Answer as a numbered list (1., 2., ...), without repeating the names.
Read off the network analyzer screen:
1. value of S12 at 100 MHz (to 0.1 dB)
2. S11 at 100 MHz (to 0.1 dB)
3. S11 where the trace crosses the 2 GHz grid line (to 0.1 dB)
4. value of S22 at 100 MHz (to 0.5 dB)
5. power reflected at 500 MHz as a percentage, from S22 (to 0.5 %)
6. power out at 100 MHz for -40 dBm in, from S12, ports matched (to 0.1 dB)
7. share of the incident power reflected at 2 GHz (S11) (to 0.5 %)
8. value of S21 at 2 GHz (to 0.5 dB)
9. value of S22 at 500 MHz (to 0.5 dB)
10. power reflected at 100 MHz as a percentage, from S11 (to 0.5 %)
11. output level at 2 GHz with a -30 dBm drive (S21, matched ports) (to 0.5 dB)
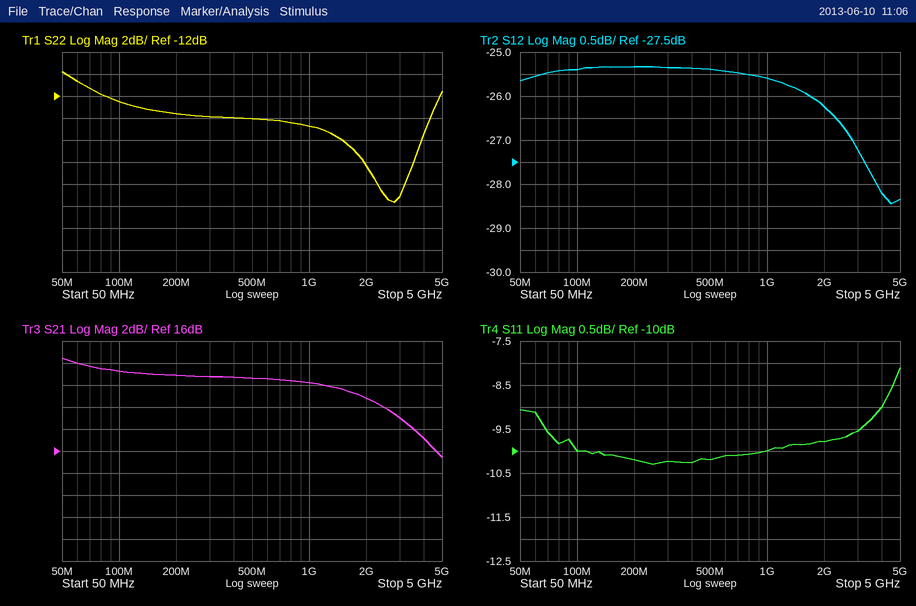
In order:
1. -25.4 dB
2. -10.0 dB
3. -9.8 dB
4. -12.5 dB
5. 4.0 %
6. -65.4 dBm
7. 10.5 %
8. 21.0 dB
9. -14.0 dB
10. 10.0 %
11. -9.0 dBm
